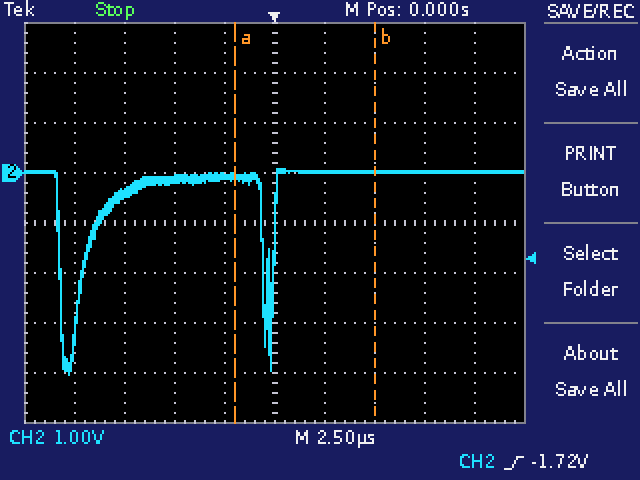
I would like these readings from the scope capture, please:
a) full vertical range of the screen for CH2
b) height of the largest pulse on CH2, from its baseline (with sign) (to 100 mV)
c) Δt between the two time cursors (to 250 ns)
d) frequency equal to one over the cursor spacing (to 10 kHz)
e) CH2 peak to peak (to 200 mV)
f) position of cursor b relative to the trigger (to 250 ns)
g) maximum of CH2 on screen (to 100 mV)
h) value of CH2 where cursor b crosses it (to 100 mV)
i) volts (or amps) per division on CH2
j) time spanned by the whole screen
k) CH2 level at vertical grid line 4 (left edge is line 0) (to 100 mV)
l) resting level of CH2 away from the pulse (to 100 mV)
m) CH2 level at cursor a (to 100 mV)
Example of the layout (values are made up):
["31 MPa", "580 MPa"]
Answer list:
["8 V", "-4.1 V", "7.00 µs", "140 kHz", "4.2 V", "+5.00 µs", "100 mV", "0.0 V", "1 V", "25 µs", "-100 mV", "0.0 V", "-100 mV"]
